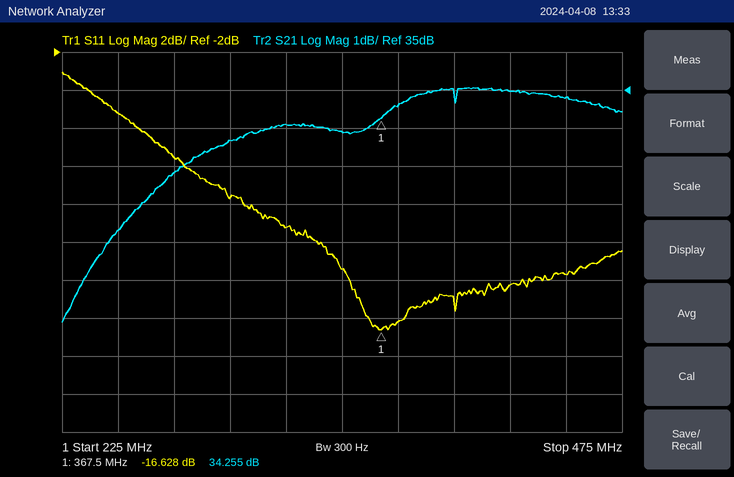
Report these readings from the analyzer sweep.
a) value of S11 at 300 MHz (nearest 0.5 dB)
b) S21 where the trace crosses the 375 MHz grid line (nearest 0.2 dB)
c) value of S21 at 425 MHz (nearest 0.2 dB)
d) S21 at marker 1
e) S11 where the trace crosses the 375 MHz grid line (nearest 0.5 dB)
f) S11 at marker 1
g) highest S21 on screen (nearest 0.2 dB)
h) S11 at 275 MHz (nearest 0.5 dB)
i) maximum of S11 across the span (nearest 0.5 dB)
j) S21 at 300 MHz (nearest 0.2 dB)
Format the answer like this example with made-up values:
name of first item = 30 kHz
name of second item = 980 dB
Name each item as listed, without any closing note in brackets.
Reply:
value of S11 at 300 MHz = -9.5 dB
S21 where the trace crosses the 375 MHz grid line = 34.6 dB
value of S21 at 425 MHz = 35.0 dB
S21 at marker 1 = 34.255 dB
S11 where the trace crosses the 375 MHz grid line = -16.0 dB
S11 at marker 1 = -16.628 dB
highest S21 on screen = 35.0 dB
S11 at 275 MHz = -7.5 dB
maximum of S11 across the span = -3.0 dB
S21 at 300 MHz = 33.6 dB
